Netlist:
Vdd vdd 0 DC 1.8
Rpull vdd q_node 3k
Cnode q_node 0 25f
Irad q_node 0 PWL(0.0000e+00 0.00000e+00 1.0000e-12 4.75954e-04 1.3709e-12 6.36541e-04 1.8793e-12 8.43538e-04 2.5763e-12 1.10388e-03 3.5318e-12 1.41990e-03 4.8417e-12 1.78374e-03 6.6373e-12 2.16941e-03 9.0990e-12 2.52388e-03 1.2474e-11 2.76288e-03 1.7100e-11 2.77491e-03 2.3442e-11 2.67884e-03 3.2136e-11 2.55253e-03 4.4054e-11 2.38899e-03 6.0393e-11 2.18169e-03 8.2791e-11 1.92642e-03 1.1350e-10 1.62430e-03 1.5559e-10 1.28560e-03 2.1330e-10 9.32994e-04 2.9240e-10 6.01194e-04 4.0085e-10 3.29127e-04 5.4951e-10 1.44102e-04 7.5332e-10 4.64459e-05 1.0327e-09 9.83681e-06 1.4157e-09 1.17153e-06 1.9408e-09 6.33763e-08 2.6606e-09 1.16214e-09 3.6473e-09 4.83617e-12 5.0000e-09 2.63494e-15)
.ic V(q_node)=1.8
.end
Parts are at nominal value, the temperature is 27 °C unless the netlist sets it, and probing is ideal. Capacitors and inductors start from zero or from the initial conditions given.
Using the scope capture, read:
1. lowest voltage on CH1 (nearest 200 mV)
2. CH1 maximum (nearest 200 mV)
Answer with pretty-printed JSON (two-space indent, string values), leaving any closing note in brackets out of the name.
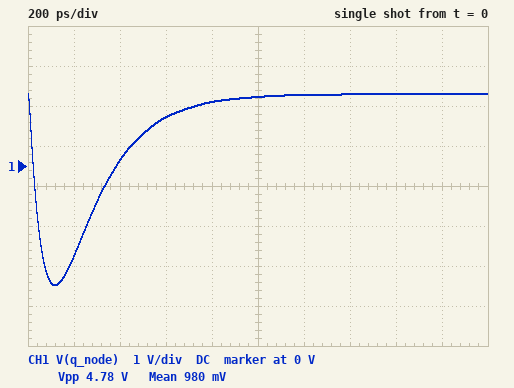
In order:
{
  "lowest voltage on CH1": "-3.0 V",
  "CH1 maximum": "1.8 V"
}
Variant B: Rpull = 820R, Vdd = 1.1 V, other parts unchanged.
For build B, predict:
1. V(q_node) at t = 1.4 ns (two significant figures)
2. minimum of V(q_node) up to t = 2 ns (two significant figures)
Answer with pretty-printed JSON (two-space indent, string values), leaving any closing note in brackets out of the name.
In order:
{
  "V(q_node) at t = 1.4 ns": "1.1 V",
  "minimum of V(q_node) up to t = 2 ns": "-700 mV"
}
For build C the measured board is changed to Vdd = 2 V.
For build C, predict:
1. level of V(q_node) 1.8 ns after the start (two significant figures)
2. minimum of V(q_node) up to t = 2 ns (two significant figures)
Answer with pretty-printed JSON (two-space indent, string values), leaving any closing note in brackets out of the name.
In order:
{
  "level of V(q_node) 1.8 ns after the start": "2.0 V",
  "minimum of V(q_node) up to t = 2 ns": "-2.8 V"
}
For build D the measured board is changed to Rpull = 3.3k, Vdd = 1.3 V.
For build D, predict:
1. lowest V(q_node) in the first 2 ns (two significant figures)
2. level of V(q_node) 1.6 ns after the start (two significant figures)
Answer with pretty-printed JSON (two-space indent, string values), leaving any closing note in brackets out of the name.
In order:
{
  "lowest V(q_node) in the first 2 ns": "-3.7 V",
  "level of V(q_node) 1.6 ns after the start": "1.3 V"
}
